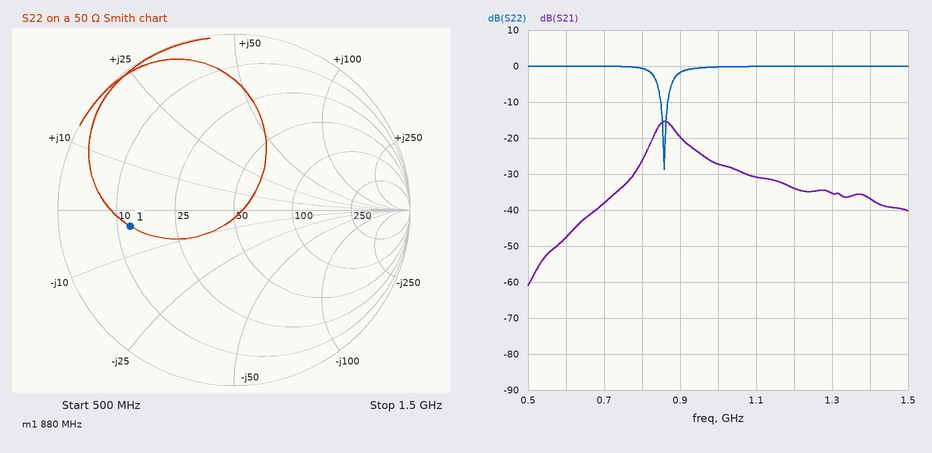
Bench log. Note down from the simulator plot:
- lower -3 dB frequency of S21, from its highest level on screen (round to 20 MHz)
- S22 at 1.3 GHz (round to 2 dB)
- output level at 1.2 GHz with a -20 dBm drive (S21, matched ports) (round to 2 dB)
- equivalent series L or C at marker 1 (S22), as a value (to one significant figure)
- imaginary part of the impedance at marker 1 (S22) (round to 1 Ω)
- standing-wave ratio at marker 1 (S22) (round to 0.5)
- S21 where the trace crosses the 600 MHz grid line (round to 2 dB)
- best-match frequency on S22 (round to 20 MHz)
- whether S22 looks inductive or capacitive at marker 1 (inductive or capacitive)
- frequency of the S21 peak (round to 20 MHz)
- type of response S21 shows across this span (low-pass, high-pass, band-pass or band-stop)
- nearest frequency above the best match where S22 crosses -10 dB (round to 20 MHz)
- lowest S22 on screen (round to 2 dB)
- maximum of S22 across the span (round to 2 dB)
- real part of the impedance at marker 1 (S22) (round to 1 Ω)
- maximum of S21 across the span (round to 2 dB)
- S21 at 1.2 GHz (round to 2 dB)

840 MHz
0 dB
-54 dBm
50 pF
-4 Ω
4.0
-48 dB
860 MHz
capacitive
860 MHz
band-pass
860 MHz
-28 dB
0 dB
13 Ω
-16 dB
-34 dB
